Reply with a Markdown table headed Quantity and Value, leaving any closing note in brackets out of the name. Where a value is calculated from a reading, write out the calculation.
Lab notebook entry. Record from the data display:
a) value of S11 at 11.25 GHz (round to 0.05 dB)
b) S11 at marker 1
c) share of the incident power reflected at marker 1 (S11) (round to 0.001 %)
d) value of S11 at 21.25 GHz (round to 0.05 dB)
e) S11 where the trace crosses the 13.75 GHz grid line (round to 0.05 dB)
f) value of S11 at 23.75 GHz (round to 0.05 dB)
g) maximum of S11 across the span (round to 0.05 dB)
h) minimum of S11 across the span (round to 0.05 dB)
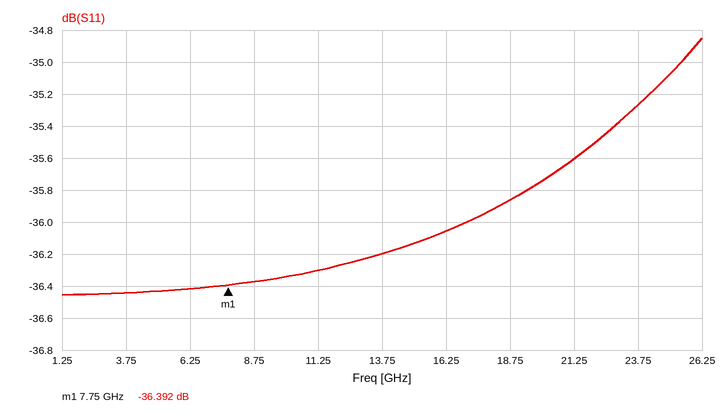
| Quantity | Value |
|---|---|
| value of S11 at 11.25 GHz | -36.30 dB |
| S11 at marker 1 | -36.392 dB |
| share of the incident power reflected at marker 1 (S11) | 10^(-36.392/10) ≈ 0.023 % |
| value of S11 at 21.25 GHz | -35.60 dB |
| S11 where the trace crosses the 13.75 GHz grid line | -36.20 dB |
| value of S11 at 23.75 GHz | -35.25 dB |
| maximum of S11 across the span | -34.85 dB |
| minimum of S11 across the span | -36.45 dB |
